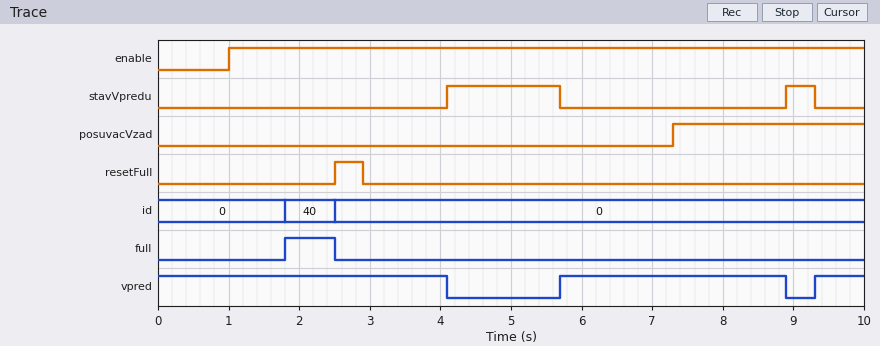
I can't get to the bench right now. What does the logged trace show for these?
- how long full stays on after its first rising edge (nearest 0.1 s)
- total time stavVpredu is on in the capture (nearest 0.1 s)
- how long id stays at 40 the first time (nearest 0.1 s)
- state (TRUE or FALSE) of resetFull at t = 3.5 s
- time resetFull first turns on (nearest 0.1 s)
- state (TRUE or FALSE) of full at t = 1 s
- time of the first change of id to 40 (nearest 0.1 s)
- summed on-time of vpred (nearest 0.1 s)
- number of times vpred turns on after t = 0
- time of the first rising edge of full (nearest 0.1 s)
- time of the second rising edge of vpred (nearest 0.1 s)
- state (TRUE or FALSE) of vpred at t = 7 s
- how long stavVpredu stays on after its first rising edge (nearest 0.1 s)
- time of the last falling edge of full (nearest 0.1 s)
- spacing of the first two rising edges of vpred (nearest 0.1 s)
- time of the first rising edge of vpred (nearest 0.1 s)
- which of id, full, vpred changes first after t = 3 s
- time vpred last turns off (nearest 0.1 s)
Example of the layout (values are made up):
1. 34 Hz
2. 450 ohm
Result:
1. 0.7 s
2. 2.0 s
3. 0.7 s
4. FALSE
5. 2.5 s
6. FALSE
7. 1.8 s
8. 8.0 s
9. 2
10. 1.8 s
11. 9.3 s
12. TRUE
13. 1.6 s
14. 2.5 s
15. 3.6 s
16. 5.7 s
17. vpred
18. 8.9 s
